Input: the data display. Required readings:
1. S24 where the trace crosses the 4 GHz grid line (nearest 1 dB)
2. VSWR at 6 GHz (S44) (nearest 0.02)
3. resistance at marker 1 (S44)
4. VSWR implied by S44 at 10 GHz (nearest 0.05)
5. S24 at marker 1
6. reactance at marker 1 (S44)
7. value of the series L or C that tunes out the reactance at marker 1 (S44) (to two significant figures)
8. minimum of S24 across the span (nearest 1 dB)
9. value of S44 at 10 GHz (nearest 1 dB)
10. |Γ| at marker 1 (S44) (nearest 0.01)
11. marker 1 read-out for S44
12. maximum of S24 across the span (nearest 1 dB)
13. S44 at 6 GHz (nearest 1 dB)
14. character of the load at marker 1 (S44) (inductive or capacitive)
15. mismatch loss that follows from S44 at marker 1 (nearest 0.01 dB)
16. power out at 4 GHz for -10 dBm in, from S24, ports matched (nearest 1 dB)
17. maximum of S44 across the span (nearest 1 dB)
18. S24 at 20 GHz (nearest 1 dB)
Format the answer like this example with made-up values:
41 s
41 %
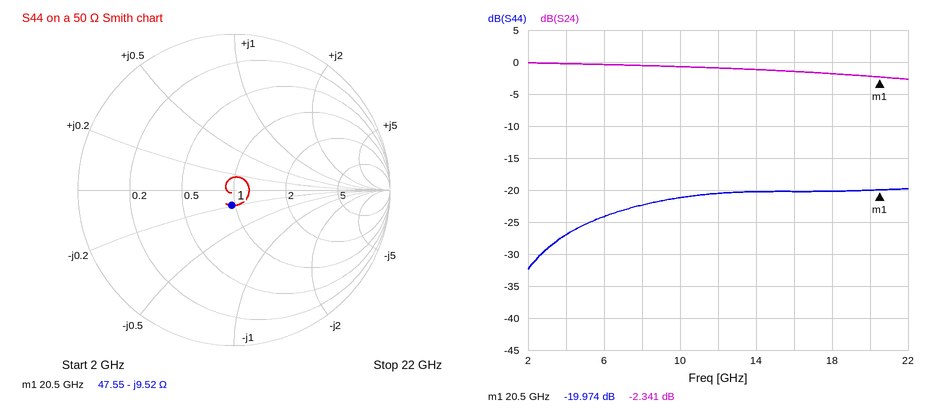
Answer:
0 dB
1.14
47.55 Ω
1.20
-2.341 dB
-9.52 Ω
74 pH
-3 dB
-21 dB
0.10
-19.974 dB
0 dB
-24 dB
capacitive
0.04 dB
-10 dBm
-20 dB
-2 dB
